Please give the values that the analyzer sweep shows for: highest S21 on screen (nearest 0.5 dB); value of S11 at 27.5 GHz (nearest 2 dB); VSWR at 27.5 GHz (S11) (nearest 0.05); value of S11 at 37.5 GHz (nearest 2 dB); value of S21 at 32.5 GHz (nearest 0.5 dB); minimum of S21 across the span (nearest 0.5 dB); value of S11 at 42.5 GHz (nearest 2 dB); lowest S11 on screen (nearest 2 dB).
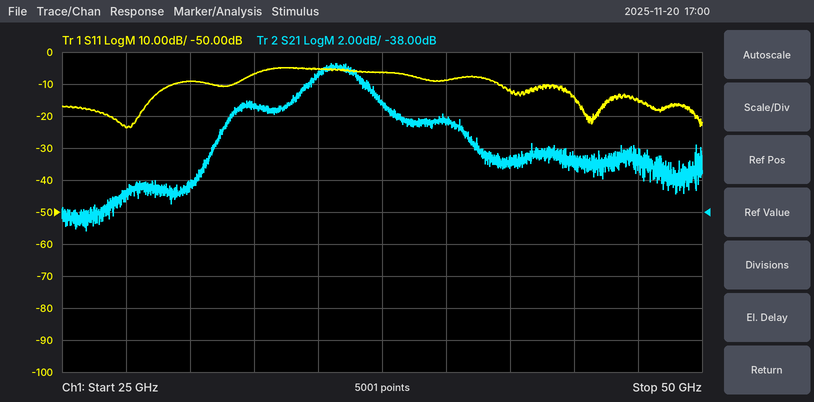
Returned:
-28.5 dB
-24 dB
1.15
-6 dB
-31.5 dB
-39.0 dB
-12 dB
-24 dB
